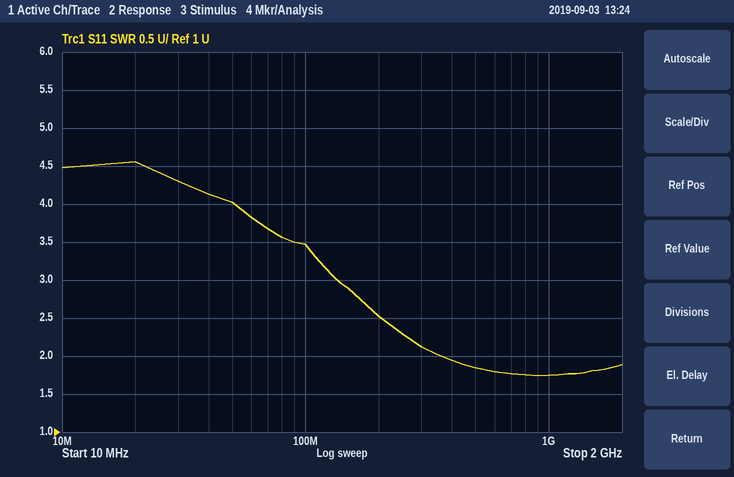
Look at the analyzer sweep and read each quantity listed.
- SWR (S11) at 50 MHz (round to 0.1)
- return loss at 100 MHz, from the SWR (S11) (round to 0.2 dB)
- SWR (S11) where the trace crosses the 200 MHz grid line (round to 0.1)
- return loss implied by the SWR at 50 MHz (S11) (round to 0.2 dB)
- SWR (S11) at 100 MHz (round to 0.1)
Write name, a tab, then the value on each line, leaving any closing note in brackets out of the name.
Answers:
SWR (S11) at 50 MHz	4.0
return loss at 100 MHz, from the SWR (S11)	5.2 dB
SWR (S11) where the trace crosses the 200 MHz grid line	2.5
return loss implied by the SWR at 50 MHz (S11)	4.4 dB
SWR (S11) at 100 MHz	3.5
